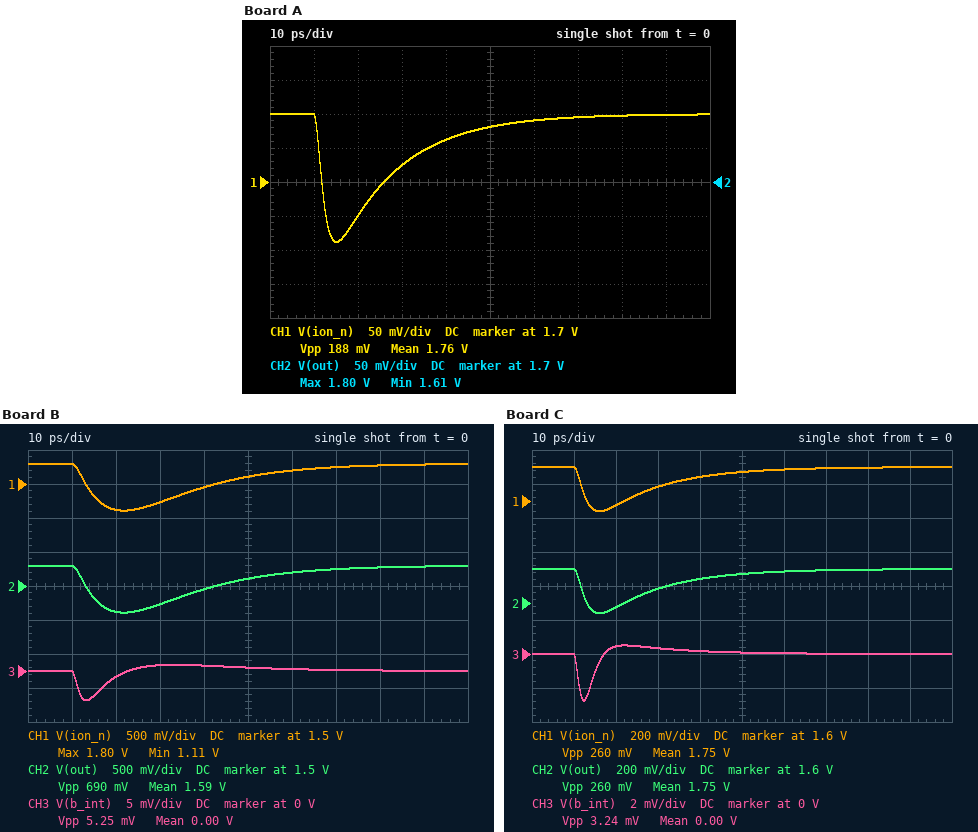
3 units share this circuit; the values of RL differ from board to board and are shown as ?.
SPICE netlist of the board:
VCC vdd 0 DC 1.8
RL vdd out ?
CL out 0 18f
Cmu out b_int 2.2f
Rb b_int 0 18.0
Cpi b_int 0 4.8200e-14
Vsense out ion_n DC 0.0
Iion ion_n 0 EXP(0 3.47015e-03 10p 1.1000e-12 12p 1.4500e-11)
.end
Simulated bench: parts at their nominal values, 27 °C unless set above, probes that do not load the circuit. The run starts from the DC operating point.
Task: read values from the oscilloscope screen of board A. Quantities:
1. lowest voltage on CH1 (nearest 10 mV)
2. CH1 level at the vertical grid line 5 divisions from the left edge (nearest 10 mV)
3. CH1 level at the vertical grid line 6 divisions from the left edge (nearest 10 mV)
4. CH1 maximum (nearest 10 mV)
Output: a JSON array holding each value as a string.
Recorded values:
["1.61 V", "1.78 V", "1.79 V", "1.80 V"]
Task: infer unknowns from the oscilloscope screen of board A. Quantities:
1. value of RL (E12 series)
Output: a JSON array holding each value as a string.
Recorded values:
["68 Ω"]
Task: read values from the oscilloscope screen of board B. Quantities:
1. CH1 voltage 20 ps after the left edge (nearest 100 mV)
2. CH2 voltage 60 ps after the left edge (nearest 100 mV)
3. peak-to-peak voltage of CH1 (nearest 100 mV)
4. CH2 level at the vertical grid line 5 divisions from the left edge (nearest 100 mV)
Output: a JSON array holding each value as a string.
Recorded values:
["1.1 V", "1.7 V", "700 mV", "1.6 V"]
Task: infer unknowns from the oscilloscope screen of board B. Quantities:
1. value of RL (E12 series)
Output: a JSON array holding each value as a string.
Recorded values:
["390 Ω"]
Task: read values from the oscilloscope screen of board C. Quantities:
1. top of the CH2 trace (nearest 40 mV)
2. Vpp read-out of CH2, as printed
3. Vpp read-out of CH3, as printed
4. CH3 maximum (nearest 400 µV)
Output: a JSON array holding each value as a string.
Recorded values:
["1.80 V", "260 mV", "3.24 mV", "400 µV"]
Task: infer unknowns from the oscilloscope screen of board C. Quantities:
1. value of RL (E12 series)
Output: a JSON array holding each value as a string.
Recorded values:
["100 Ω"]
